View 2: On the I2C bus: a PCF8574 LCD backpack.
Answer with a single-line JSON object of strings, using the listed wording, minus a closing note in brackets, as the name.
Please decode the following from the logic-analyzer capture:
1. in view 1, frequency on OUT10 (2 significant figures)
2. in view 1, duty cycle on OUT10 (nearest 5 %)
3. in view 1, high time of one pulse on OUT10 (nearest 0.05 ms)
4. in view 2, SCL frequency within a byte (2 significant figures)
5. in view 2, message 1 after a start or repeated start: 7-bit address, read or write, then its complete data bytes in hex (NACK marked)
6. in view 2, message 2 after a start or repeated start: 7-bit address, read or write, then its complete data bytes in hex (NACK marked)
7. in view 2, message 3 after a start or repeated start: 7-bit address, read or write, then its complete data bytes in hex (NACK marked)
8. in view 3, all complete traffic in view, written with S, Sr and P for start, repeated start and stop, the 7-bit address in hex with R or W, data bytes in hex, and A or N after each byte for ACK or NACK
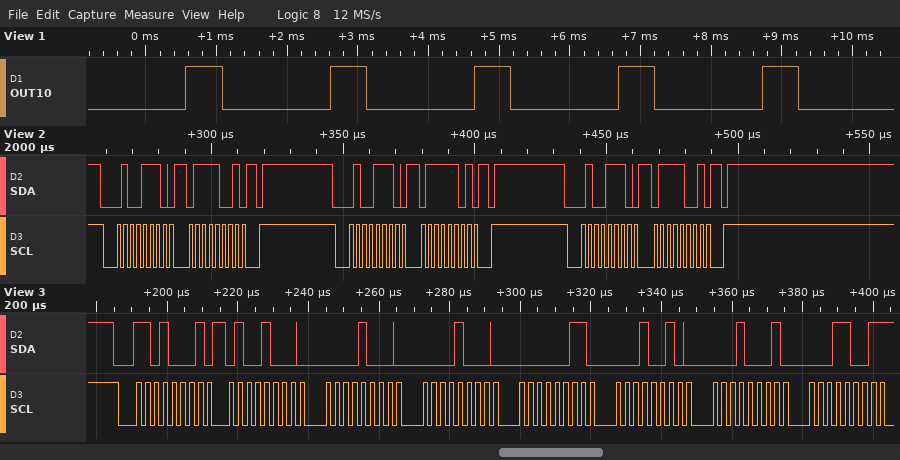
{"in view 1, frequency on OUT10": "490 Hz", "in view 1, duty cycle on OUT10": "25 %", "in view 1, high time of one pulse on OUT10": "0.50 ms", "in view 2, SCL frequency within a byte": "400 kHz", "in view 2, message 1 after a start or repeated start: 7-bit address, read or write, then its complete data bytes in hex": "0x27 write: 79", "in view 2, message 2 after a start or repeated start: 7-bit address, read or write, then its complete data bytes in hex": "0x27 write: 7D", "in view 2, message 3 after a start or repeated start: 7-bit address, read or write, then its complete data bytes in hex": "0x27 write: 79", "in view 3, all complete traffic in view, written with S, Sr and P for start, repeated start and stop, the 7-bit address in hex with R or W, data bytes in hex, and A or N after each byte for ACK or NACK": "S 68R A 48 A 08 A 08 A 03 A 12 A 11 A 19 N"}
